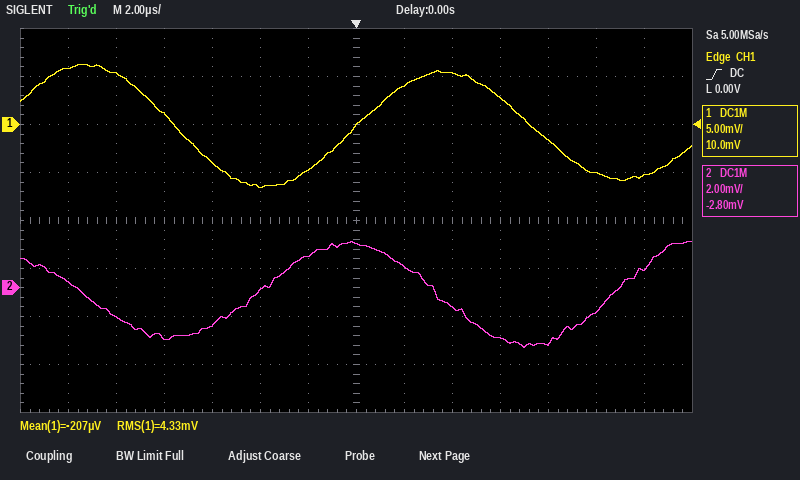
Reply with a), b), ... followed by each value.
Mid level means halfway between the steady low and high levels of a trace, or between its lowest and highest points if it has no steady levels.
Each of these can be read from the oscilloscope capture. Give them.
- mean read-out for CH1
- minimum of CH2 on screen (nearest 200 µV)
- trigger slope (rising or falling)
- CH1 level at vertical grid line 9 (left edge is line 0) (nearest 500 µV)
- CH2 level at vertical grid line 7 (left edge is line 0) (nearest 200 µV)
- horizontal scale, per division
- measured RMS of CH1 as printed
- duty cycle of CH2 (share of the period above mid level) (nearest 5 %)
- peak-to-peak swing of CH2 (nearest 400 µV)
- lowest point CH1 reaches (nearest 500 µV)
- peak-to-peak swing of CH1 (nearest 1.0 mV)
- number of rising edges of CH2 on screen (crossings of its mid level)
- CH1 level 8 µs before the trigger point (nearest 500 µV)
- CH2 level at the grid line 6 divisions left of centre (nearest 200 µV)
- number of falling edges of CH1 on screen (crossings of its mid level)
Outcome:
a) -207 µV
b) -2.4 mV
c) rising
d) 5.5 mV
e) 1.8 mV
f) 2 µs
g) 4.33 mV
h) 50 %
i) 4.4 mV
j) -6.5 mV
k) 13.0 mV
l) 2
m) 1.0 mV
n) 200 µV
o) 2
